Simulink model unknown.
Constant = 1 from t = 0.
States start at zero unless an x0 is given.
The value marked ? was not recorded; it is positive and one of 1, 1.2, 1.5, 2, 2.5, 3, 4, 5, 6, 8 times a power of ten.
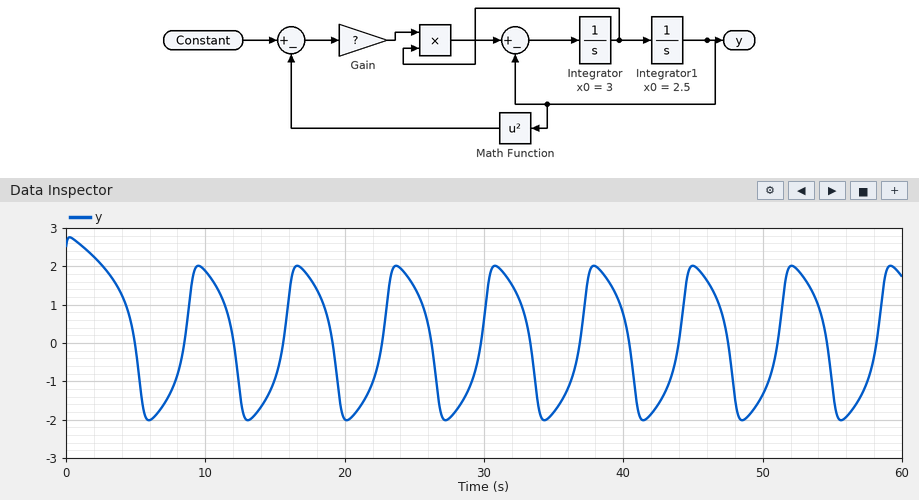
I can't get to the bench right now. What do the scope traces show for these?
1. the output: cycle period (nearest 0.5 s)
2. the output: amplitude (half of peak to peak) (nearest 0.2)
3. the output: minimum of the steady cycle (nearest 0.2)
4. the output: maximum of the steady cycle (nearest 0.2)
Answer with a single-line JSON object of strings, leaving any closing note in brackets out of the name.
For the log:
{"the output: cycle period": "7.0 s", "the output: amplitude (half of peak to peak)": "2.0", "the output: minimum of the steady cycle": "-2.0", "the output: maximum of the steady cycle": "2.0"}
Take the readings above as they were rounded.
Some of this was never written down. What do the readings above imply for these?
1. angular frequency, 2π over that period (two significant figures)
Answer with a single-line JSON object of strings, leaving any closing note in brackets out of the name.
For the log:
{"angular frequency, 2π over that period": "0.90 rad/s"}
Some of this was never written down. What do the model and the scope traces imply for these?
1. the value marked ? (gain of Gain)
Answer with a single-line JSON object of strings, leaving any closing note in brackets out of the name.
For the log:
{"the value marked ?": "1.5"}
